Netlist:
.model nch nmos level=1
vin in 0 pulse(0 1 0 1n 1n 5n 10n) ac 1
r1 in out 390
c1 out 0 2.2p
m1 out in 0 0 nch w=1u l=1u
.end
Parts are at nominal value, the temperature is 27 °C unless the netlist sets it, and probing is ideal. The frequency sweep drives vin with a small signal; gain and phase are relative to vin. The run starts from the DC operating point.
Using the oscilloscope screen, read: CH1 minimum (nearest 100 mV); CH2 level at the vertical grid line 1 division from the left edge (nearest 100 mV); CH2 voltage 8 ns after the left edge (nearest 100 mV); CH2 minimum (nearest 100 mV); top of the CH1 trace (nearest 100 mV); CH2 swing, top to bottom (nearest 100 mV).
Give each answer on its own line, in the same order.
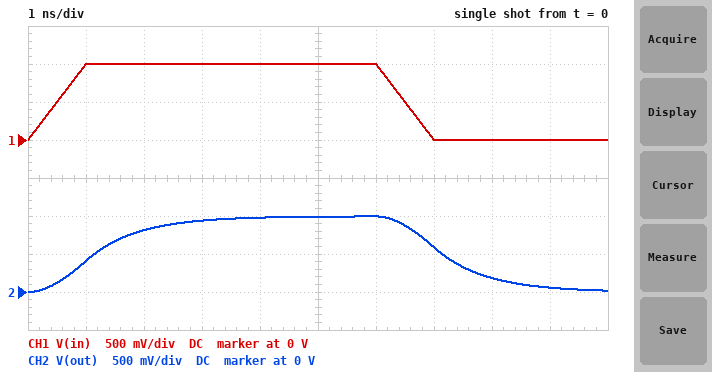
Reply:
0 V
400 mV
200 mV
0 V
1.0 V
1.0 V
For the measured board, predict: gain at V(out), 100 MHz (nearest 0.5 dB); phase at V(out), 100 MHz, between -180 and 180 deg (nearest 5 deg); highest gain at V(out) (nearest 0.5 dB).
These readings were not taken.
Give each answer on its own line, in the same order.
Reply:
-1.0 dB
-30 deg
0 dB
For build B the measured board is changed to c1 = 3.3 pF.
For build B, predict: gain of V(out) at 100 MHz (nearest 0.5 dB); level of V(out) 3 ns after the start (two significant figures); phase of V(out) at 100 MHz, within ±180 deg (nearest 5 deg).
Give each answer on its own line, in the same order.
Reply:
-2.0 dB
850 mV
-40 deg
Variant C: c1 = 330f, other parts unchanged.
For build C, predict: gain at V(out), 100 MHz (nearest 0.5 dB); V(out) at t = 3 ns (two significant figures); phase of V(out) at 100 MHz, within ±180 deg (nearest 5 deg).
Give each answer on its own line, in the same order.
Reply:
0 dB
1.0 V
-5 deg
